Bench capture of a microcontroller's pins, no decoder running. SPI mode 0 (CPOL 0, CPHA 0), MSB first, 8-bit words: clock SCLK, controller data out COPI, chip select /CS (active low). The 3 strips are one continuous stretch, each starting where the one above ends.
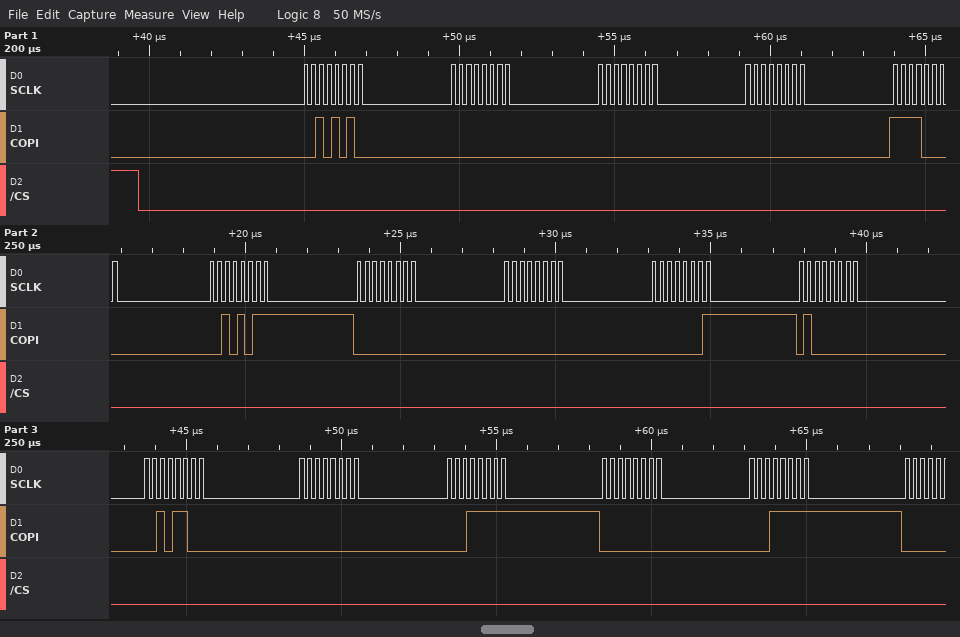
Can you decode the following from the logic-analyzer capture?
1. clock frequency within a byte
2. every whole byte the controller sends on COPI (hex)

4 MHz
0x2A 0x00 0x00 0x00 0xF0 0x2B 0x00 0x00 0x01 0x40 0x2C 0x00 0x1F 0x00 0x1F
